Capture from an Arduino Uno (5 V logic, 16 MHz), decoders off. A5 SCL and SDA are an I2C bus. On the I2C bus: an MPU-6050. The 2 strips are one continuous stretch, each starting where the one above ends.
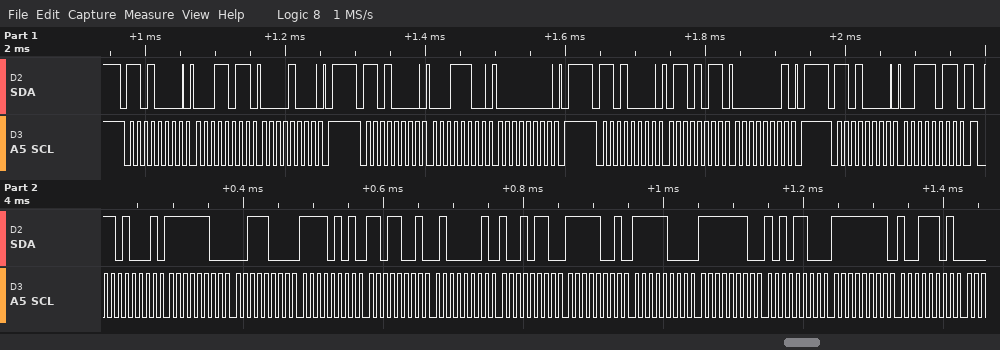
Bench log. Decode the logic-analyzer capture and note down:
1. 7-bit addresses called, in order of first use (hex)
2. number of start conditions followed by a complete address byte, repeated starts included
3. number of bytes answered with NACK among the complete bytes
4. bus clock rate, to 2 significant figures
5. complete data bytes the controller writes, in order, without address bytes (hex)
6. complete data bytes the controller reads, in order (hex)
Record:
0x68
5
0
100 kHz
1B 08 1C 00 6B 01 3B
FC 38 F5 D9 41 96 F9 F8 FE AC FF 9D
